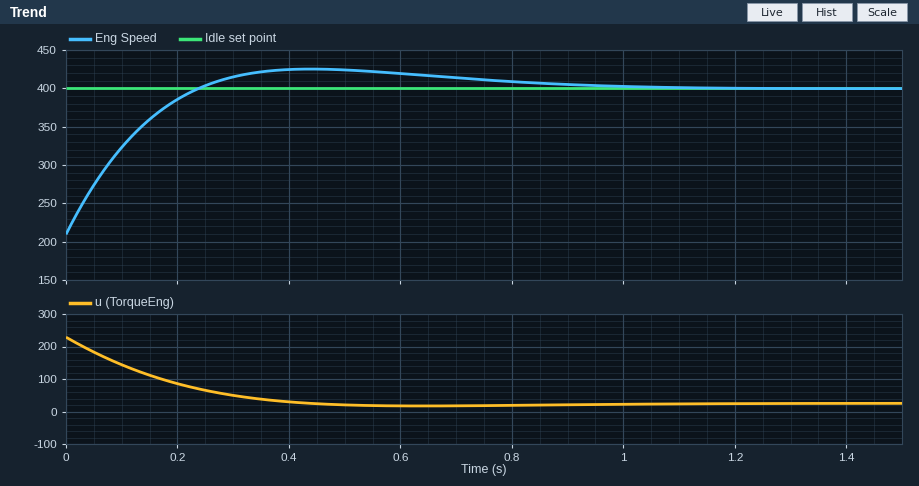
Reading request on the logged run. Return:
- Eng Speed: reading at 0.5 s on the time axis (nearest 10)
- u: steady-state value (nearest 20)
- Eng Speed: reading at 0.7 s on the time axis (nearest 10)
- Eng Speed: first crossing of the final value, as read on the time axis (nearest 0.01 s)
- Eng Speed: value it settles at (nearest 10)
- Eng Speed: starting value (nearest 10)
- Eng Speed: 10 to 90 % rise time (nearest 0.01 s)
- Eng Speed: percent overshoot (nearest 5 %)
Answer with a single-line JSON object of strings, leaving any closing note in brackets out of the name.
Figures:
{"Eng Speed: reading at 0.5 s on the time axis": "420", "u: steady-state value": "20", "Eng Speed: reading at 0.7 s on the time axis": "410", "Eng Speed: first crossing of the final value, as read on the time axis": "0.24 s", "Eng Speed: value it settles at": "400", "Eng Speed: starting value": "210", "Eng Speed: 10 to 90 % rise time": "0.18 s", "Eng Speed: percent overshoot": "15 %"}
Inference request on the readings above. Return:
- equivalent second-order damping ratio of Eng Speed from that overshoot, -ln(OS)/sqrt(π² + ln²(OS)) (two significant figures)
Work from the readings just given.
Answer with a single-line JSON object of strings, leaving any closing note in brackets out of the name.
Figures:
{"equivalent second-order damping ratio of Eng Speed from that overshoot, -ln(OS)/sqrt(π² + ln²(OS))": "0.52"}
